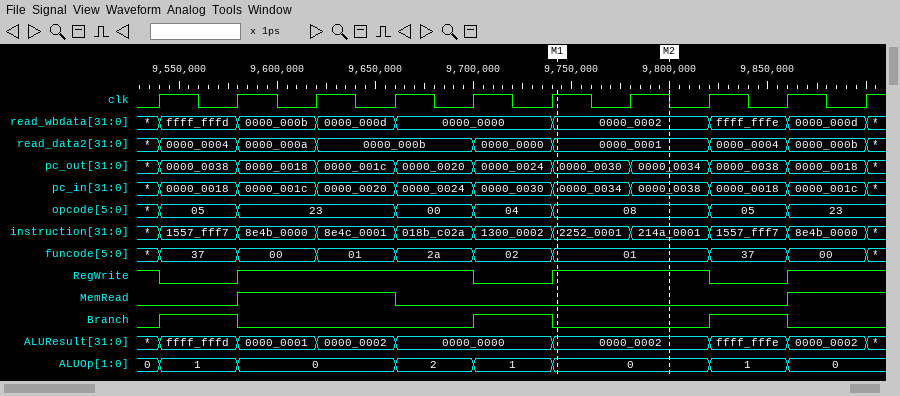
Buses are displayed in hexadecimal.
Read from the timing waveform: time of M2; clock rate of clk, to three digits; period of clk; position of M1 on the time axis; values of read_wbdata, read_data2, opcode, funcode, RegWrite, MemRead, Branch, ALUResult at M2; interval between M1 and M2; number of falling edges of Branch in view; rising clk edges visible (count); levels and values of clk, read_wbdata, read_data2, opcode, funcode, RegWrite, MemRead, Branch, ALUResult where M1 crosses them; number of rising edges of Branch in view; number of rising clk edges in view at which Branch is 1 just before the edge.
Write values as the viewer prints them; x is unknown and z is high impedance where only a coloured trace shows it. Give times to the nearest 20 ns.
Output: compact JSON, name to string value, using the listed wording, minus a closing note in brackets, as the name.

{"time of M2": "9800 ns", "clock rate of clk, to three digits": "25.0 MHz", "period of clk": "40 ns", "position of M1 on the time axis": "9740 ns", "values of read_wbdata, read_data2, opcode, funcode, RegWrite, MemRead, Branch, ALUResult at M2": "read_wbdata=0000_0002, read_data2=0000_0001, opcode=08, funcode=01, RegWrite=1, MemRead=0, Branch=0, ALUResult=0000_0002", "interval between M1 and M2": "60 ns", "number of falling edges of Branch in view": "3", "rising clk edges visible": "10", "levels and values of clk, read_wbdata, read_data2, opcode, funcode, RegWrite, MemRead, Branch, ALUResult where M1 crosses them": "clk=1, read_wbdata=0000_0002, read_data2=0000_0001, opcode=08, funcode=01, RegWrite=1, MemRead=0, Branch=0, ALUResult=0000_0002", "number of rising edges of Branch in view": "3", "number of rising clk edges in view at which Branch is 1 just before the edge": "3"}
